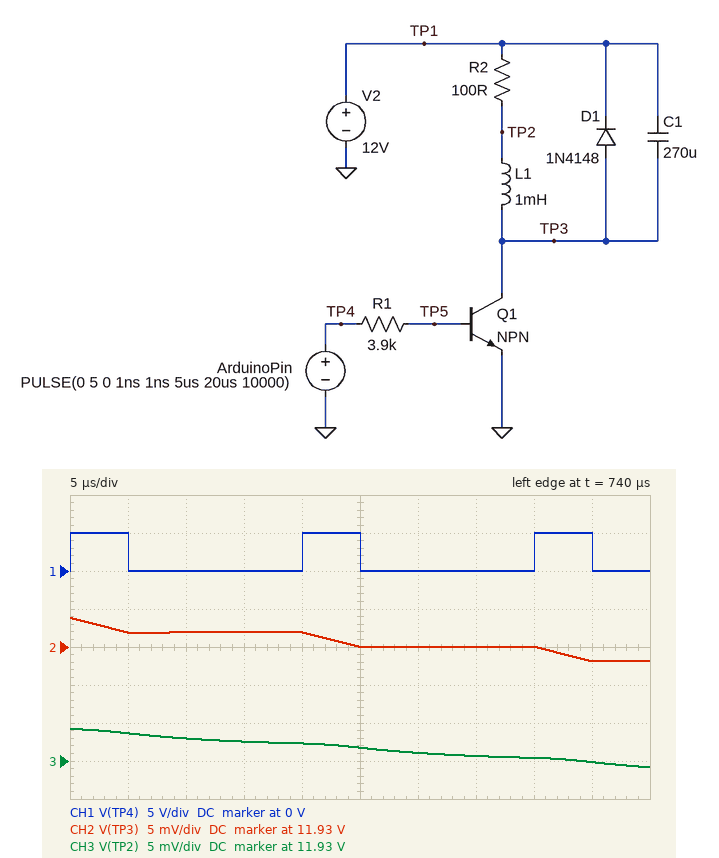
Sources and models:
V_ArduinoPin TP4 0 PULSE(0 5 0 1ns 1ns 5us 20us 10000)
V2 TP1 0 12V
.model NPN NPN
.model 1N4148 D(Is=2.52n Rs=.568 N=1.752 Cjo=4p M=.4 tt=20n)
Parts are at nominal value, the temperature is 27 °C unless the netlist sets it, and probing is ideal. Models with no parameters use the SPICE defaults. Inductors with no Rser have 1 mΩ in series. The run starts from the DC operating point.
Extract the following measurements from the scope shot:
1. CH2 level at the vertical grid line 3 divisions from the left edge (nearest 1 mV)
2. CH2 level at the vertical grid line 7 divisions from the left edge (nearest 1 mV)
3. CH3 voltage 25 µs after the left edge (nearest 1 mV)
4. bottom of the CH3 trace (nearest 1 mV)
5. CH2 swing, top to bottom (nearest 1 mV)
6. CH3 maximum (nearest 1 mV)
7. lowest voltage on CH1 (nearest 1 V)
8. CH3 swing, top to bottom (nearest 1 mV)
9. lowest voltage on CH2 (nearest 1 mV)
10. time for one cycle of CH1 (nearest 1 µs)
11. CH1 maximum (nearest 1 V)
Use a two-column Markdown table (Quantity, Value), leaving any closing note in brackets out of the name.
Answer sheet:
| Quantity | Value |
|---|---|
| CH2 level at the vertical grid line 3 divisions from the left edge | 11.927 V |
| CH2 level at the vertical grid line 7 divisions from the left edge | 11.925 V |
| CH3 voltage 25 µs after the left edge | 11.927 V |
| bottom of the CH3 trace | 11.924 V |
| CH2 swing, top to bottom | 6 mV |
| CH3 maximum | 11.929 V |
| lowest voltage on CH1 | 0 V |
| CH3 swing, top to bottom | 5 mV |
| lowest voltage on CH2 | 11.923 V |
| time for one cycle of CH1 | 20 µs |
| CH1 maximum | 5 V |
